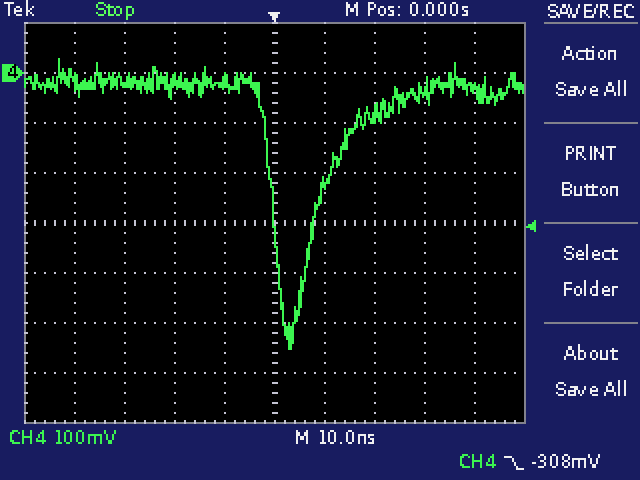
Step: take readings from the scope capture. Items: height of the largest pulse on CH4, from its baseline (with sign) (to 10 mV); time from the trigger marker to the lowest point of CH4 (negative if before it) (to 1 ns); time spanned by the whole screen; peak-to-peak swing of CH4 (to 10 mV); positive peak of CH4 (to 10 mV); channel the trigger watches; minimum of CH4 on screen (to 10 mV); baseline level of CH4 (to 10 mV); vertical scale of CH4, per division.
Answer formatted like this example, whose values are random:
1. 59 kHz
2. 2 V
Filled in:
1. -530 mV
2. +3 ns
3. 100 ns
4. 580 mV
5. 30 mV
6. CH4
7. -550 mV
8. -20 mV
9. 100 mV
